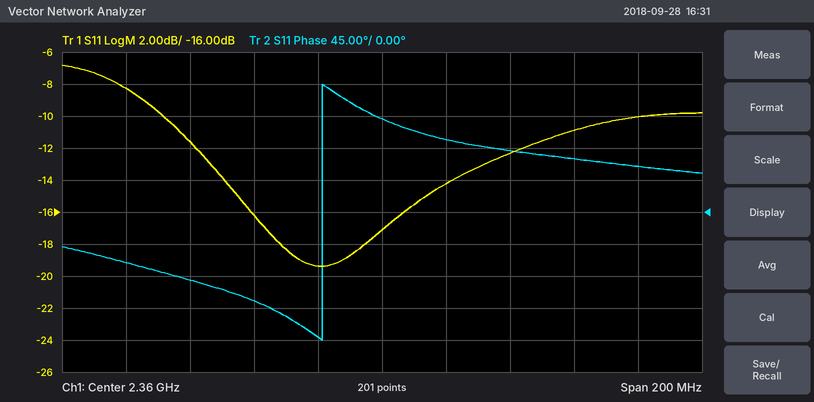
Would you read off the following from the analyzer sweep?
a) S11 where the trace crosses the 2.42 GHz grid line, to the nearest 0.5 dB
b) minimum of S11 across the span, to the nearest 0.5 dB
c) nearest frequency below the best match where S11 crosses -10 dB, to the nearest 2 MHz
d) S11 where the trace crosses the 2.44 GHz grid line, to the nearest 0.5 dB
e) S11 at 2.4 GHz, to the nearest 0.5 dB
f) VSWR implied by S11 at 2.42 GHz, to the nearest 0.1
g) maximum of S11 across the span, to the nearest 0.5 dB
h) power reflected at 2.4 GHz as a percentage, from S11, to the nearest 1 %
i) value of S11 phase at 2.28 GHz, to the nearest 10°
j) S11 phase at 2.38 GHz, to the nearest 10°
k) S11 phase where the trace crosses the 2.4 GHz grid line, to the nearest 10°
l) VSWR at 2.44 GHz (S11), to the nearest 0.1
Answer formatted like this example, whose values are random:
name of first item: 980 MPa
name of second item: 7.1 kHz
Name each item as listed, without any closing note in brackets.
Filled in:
S11 where the trace crosses the 2.42 GHz grid line, to the nearest 0.5 dB: -11.0 dB
minimum of S11 across the span, to the nearest 0.5 dB: -19.5 dB
nearest frequency below the best match where S11 crosses -10 dB, to the nearest 2 MHz: 2.292 GHz
S11 where the trace crosses the 2.44 GHz grid line, to the nearest 0.5 dB: -10.0 dB
S11 at 2.4 GHz, to the nearest 0.5 dB: -12.5 dB
VSWR implied by S11 at 2.42 GHz, to the nearest 0.1: 1.8
maximum of S11 across the span, to the nearest 0.5 dB: -7.0 dB
power reflected at 2.4 GHz as a percentage, from S11, to the nearest 1 %: 6 %
value of S11 phase at 2.28 GHz, to the nearest 10°: -70°
S11 phase at 2.38 GHz, to the nearest 10°: 100°
S11 phase where the trace crosses the 2.4 GHz grid line, to the nearest 10°: 90°
VSWR at 2.44 GHz (S11), to the nearest 0.1: 1.9
